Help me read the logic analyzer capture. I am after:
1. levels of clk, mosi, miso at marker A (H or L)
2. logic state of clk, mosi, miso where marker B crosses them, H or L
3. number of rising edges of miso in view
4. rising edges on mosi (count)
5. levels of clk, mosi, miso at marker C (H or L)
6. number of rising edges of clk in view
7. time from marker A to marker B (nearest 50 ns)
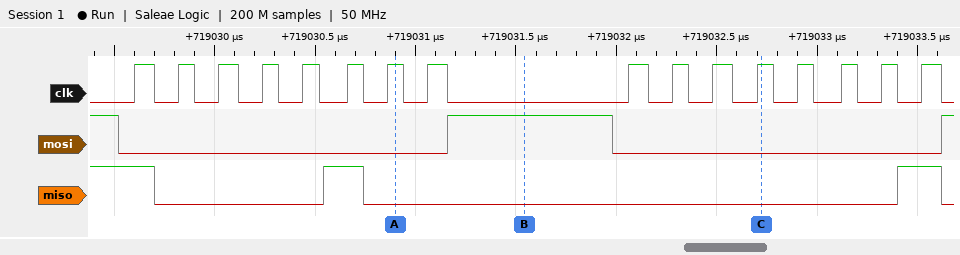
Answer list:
clk=H, mosi=L, miso=L
clk=L, mosi=H, miso=L
2
2
clk=H, mosi=L, miso=L
16
650 ns
